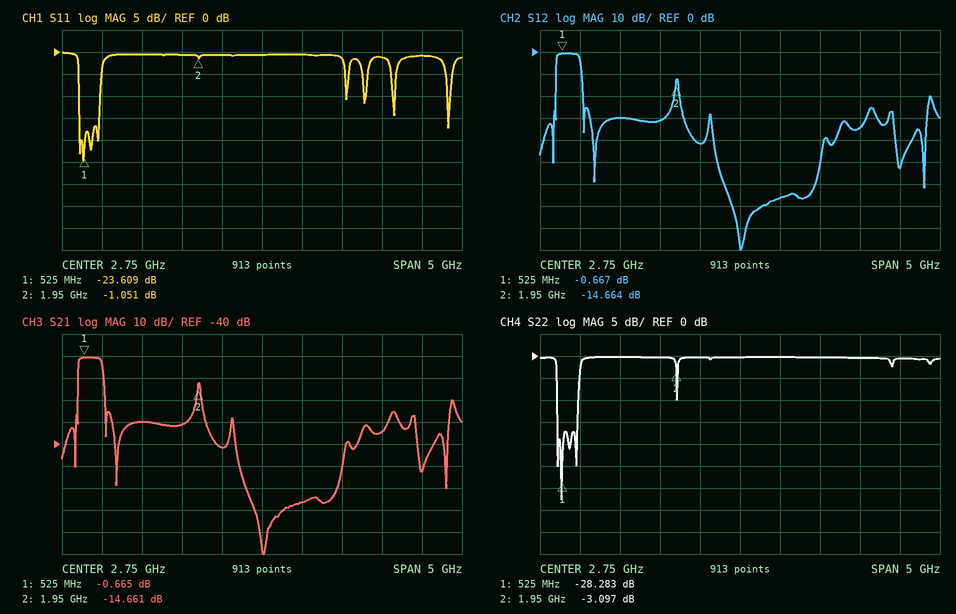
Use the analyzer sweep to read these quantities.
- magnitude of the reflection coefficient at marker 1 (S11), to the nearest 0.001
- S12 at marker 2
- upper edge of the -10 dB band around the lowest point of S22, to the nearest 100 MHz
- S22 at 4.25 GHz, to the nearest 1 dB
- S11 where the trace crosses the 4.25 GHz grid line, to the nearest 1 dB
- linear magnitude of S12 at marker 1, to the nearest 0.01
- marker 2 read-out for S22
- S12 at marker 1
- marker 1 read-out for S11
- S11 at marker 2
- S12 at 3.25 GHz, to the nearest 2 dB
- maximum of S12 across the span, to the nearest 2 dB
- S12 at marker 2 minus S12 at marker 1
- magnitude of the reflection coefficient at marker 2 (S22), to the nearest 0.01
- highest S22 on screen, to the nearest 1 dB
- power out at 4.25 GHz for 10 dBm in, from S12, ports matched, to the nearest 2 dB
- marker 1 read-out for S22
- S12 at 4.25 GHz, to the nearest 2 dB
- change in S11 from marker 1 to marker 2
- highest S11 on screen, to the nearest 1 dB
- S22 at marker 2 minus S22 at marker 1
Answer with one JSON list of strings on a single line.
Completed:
["0.066", "-14.664 dB", "700 MHz", "0 dB", "-1 dB", "0.93", "-3.097 dB", "-0.667 dB", "-23.609 dB", "-1.051 dB", "-66 dB", "0 dB", "-13.997 dB", "0.70", "0 dB", "-24 dBm", "-28.283 dB", "-34 dB", "22.558 dB", "0 dB", "25.186 dB"]
